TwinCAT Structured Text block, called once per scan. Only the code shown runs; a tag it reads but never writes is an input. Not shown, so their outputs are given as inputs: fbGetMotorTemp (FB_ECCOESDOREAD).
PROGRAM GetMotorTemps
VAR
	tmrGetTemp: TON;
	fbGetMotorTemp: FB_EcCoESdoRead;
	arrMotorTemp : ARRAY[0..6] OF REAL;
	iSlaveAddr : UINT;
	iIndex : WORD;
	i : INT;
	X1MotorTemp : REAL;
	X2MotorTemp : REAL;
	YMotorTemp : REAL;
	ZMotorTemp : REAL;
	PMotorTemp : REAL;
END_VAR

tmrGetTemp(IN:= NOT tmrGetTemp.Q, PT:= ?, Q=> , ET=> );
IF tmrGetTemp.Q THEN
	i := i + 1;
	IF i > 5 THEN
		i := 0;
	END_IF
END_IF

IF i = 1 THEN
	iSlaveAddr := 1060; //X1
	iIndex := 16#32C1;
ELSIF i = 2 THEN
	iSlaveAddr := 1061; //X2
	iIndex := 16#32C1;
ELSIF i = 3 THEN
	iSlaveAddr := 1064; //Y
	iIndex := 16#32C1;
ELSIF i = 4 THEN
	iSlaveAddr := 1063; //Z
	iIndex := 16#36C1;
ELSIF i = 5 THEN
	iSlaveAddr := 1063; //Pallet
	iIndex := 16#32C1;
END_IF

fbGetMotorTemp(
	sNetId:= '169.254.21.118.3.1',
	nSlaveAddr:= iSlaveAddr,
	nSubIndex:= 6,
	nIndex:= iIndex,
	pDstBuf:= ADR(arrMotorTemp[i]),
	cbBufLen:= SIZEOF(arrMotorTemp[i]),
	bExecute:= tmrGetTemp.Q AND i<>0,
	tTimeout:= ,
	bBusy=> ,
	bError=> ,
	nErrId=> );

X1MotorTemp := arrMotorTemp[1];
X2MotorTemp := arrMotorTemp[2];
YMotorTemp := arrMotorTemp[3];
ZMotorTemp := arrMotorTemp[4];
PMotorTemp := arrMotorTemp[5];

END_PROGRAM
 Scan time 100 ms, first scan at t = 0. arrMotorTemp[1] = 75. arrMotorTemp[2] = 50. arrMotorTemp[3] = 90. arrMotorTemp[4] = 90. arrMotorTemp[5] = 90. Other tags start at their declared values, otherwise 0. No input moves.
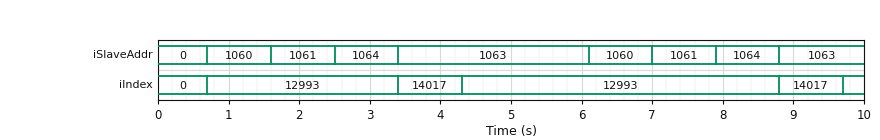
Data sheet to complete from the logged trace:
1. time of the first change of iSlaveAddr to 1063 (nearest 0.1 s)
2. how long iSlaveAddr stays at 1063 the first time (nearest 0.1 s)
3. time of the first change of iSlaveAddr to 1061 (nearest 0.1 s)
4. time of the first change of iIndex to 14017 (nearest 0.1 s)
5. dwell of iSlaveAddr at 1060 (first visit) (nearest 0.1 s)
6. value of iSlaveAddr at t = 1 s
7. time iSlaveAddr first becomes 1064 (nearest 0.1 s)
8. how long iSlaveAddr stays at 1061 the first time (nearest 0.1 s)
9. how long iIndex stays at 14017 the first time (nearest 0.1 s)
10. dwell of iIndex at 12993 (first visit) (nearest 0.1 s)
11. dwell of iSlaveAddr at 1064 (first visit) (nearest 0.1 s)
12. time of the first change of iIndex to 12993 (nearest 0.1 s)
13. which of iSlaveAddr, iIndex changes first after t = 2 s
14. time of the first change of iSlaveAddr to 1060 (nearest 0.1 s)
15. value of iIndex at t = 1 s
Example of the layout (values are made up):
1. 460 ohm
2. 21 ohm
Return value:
1. 3.4 s
2. 2.7 s
3. 1.6 s
4. 3.4 s
5. 0.9 s
6. 1060
7. 2.5 s
8. 0.9 s
9. 0.9 s
10. 2.7 s
11. 0.9 s
12. 0.7 s
13. iSlaveAddr
14. 0.7 s
15. 12993
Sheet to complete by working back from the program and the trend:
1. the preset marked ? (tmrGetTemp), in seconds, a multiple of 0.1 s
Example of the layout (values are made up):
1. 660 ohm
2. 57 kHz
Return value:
1. 0.7 s
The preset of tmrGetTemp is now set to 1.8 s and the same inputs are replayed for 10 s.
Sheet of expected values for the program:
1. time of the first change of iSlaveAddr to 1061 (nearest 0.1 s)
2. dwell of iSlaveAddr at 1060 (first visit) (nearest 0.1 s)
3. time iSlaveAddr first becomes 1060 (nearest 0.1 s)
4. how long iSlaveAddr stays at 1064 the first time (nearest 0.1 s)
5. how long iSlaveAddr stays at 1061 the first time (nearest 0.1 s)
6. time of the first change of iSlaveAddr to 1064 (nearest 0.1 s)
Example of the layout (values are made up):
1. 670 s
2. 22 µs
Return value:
1. 3.8 s
2. 2.0 s
3. 1.8 s
4. 2.0 s
5. 2.0 s
6. 5.8 s
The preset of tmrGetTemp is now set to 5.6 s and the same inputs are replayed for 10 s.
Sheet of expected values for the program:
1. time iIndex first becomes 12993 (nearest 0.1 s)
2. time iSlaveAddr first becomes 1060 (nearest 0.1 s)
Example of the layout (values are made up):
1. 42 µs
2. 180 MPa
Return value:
1. 5.6 s
2. 5.6 s
